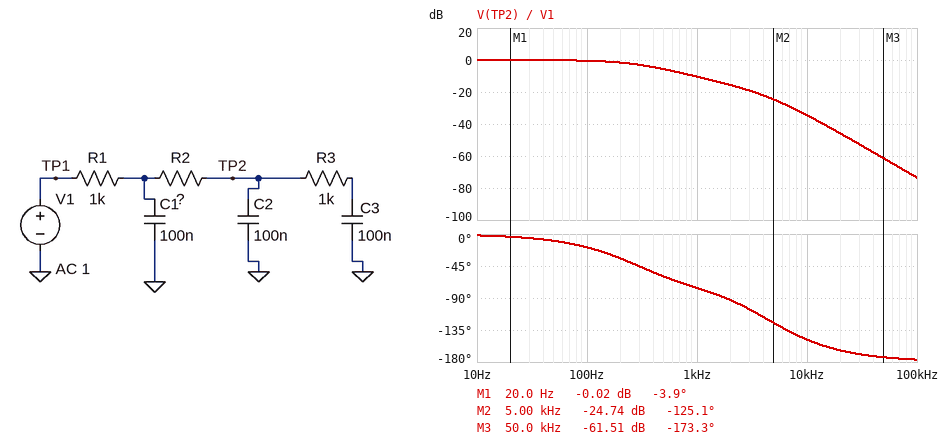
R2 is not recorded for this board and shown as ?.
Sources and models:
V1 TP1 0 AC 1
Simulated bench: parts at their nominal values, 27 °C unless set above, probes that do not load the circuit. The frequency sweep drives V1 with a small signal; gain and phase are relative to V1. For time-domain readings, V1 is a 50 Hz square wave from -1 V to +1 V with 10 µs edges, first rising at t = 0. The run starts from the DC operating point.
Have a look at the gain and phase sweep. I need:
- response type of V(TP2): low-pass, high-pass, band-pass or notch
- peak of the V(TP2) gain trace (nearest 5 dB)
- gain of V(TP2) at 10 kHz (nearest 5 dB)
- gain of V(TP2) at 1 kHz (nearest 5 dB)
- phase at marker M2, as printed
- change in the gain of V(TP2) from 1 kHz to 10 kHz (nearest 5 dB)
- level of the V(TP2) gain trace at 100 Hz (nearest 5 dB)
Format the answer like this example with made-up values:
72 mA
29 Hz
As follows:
low-pass
0 dB
-35 dB
-10 dB
-125.1 deg
-25 dB
0 dB
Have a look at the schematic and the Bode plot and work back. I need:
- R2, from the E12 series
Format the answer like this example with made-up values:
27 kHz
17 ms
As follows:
1.2 kΩ
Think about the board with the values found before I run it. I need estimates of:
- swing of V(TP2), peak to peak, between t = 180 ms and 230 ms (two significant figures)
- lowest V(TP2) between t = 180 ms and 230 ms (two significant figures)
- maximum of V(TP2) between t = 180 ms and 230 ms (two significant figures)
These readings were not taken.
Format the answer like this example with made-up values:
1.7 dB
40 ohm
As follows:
2.0 V
-1.0 V
1.0 V
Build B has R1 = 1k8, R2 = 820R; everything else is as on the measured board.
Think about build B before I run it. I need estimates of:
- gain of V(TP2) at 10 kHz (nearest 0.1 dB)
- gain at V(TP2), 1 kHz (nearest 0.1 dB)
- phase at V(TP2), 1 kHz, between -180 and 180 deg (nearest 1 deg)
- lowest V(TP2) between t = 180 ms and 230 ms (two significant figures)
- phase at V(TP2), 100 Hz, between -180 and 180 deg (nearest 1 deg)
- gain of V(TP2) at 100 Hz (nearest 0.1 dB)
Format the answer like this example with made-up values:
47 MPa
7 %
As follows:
-36.6 dB
-12.6 dB
-80 deg
-1.0 V
-24 deg
-0.8 dB
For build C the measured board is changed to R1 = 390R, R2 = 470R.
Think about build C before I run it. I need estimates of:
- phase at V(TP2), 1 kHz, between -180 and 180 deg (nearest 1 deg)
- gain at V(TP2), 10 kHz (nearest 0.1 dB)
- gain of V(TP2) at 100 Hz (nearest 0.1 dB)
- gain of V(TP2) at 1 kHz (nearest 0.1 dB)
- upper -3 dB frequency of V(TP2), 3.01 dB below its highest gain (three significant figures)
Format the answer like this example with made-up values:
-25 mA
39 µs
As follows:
-47 deg
-20.6 dB
-0.1 dB
-4.3 dB
730 Hz
